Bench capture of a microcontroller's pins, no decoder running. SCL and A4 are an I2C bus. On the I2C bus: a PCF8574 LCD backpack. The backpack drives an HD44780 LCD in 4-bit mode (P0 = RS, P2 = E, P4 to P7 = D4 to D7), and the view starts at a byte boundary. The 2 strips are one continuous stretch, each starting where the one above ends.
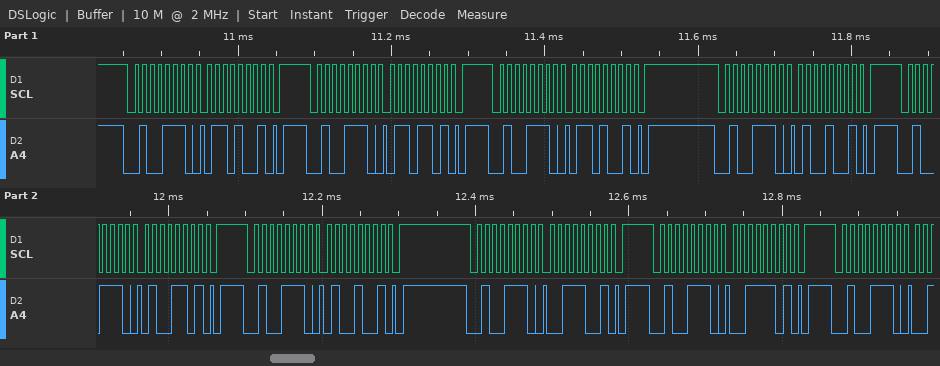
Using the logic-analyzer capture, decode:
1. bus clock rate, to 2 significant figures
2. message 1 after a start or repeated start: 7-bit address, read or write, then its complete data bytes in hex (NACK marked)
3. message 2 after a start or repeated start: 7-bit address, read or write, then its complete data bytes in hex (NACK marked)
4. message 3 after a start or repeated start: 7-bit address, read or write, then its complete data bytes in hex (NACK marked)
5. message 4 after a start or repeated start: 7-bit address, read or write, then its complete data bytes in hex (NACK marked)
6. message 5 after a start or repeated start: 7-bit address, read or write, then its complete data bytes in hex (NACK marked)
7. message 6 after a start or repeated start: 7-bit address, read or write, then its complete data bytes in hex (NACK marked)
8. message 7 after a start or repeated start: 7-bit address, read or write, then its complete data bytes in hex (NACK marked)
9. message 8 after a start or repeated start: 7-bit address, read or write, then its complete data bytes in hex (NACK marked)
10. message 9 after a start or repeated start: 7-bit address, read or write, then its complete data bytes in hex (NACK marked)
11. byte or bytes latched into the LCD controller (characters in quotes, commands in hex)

100 kHz
0x27 write: 69
0x27 write: 6D
0x27 write: 69
0x27 write: 49
0x27 write: 4D
0x27 write: 49
0x27 write: 39
0x27 write: 3D
0x27 write
'd'
